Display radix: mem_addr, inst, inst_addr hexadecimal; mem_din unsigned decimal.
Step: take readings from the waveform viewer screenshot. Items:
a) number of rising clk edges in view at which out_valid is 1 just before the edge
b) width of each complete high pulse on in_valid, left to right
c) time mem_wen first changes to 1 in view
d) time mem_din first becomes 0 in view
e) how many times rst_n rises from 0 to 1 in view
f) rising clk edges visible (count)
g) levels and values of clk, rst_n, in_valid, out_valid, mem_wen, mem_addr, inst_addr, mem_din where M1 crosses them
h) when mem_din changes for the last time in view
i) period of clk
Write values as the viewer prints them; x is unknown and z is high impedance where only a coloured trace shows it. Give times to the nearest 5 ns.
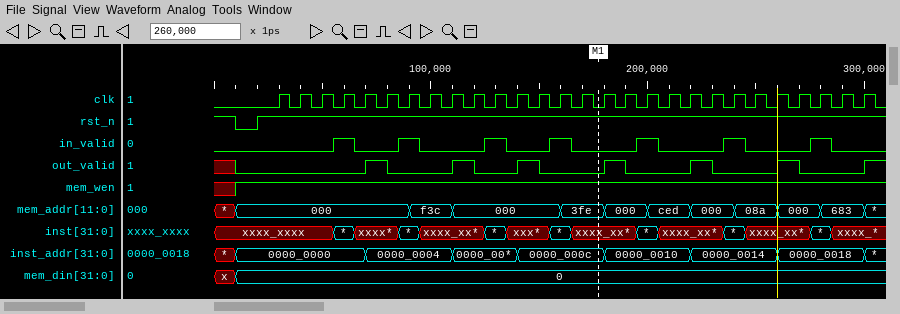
6
10 ns, 10 ns, 10 ns, 10 ns, 10 ns, 10 ns, 10 ns
10 ns
10 ns
1
28
clk=0, rst_n=1, in_valid=0, out_valid=0, mem_wen=1, mem_addr=3fe, inst_addr=0000_000c, mem_din=0
10 ns
10 ns
